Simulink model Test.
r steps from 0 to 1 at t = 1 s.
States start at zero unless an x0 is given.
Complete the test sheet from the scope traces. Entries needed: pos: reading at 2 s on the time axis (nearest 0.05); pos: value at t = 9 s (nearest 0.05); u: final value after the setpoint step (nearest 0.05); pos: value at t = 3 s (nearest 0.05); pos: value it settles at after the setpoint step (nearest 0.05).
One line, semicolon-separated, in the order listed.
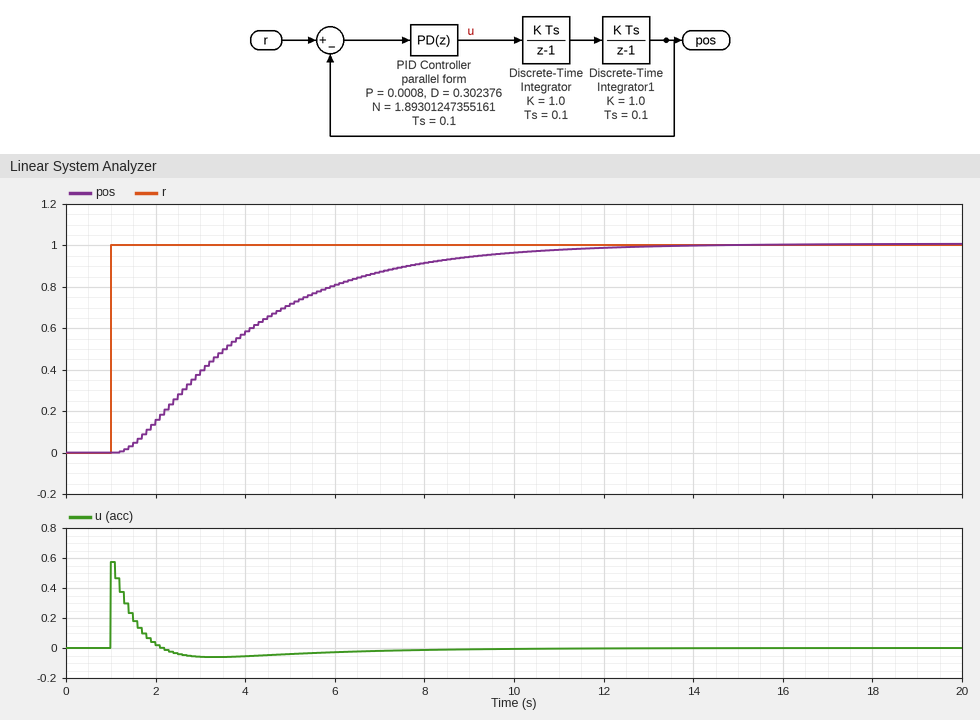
0.15; 0.95; 0.00; 0.40; 1.00
